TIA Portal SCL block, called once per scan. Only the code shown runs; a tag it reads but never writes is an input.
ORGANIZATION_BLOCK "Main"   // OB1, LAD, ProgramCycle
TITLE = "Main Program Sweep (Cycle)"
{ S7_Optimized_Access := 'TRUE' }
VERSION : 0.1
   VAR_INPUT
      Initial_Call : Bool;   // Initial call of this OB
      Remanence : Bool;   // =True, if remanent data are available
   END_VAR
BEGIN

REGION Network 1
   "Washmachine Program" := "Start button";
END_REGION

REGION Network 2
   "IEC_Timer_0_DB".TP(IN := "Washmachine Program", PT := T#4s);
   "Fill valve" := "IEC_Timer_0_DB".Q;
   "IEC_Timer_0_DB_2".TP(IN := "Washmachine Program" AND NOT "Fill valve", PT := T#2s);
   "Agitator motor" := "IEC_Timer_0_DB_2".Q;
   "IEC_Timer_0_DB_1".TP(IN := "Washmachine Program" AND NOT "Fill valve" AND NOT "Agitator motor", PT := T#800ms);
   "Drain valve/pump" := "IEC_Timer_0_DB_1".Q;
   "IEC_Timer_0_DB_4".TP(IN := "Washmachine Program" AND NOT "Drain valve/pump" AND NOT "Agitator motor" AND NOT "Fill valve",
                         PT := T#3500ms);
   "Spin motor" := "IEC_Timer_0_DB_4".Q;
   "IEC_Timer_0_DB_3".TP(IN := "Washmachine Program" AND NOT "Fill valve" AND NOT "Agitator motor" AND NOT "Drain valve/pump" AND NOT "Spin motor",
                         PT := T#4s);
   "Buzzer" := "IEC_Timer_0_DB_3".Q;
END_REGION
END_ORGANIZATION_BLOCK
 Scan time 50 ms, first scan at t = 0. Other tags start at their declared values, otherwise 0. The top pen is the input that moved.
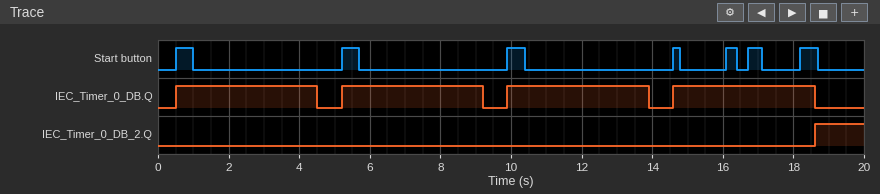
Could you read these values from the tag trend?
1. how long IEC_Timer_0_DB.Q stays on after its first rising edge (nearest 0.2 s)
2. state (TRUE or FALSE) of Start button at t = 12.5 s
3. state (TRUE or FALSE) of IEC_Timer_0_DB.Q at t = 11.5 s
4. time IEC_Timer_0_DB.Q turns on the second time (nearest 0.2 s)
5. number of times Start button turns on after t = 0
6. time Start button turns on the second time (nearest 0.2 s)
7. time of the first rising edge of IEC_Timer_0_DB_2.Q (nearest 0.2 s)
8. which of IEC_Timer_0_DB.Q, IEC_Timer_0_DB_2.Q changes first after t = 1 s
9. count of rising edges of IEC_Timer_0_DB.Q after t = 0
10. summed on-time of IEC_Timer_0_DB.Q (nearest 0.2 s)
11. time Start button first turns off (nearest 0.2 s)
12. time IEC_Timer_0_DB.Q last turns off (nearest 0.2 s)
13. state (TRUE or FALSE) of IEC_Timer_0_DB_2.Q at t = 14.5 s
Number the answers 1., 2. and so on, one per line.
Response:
1. 4.0 s
2. FALSE
3. TRUE
4. 5.2 s
5. 7
6. 5.2 s
7. 18.6 s
8. IEC_Timer_0_DB.Q
9. 4
10. 16.0 s
11. 1.0 s
12. 18.6 s
13. FALSE
